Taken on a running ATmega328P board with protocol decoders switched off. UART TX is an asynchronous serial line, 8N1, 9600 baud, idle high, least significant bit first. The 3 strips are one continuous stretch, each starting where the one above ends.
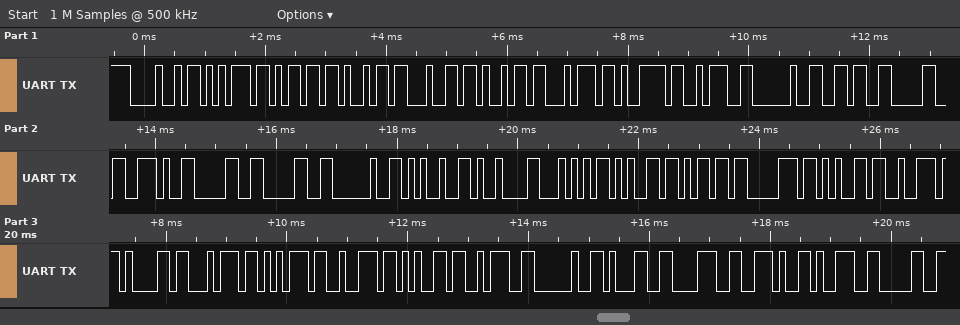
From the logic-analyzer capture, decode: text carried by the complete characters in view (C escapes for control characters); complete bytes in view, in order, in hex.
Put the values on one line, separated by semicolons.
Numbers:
"Humidity: 60.00 %\tTemperature: 18.90"; 48 75 6D 69 64 69 74 79 3A 20 36 30 2E 30 30 20 25 09 54 65 6D 70 65 72 61 74 75 72 65 3A 20 31 38 2E 39 30
